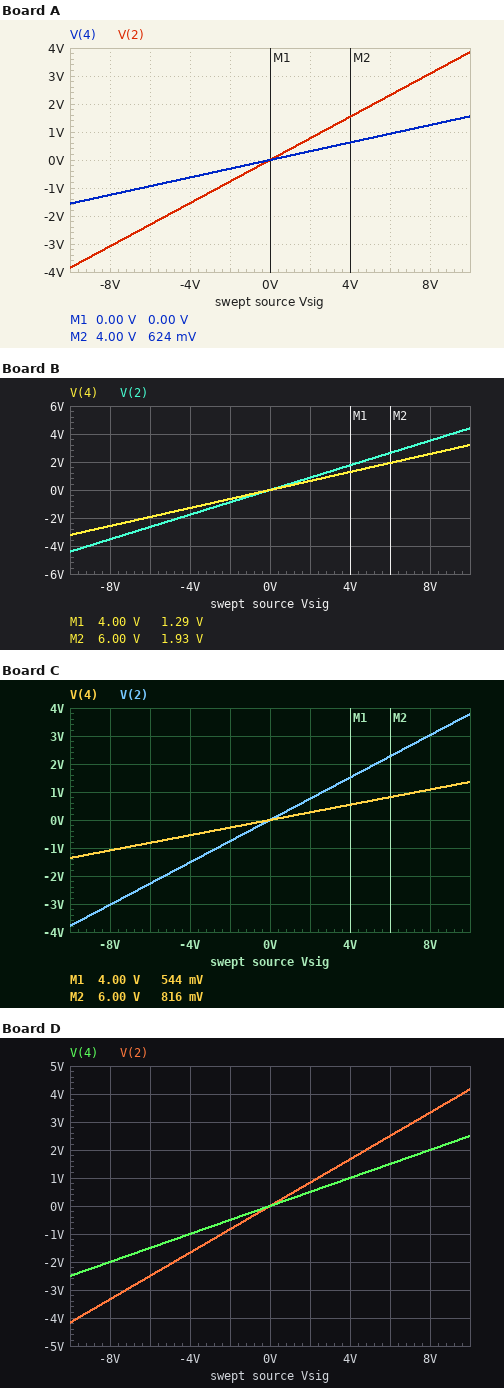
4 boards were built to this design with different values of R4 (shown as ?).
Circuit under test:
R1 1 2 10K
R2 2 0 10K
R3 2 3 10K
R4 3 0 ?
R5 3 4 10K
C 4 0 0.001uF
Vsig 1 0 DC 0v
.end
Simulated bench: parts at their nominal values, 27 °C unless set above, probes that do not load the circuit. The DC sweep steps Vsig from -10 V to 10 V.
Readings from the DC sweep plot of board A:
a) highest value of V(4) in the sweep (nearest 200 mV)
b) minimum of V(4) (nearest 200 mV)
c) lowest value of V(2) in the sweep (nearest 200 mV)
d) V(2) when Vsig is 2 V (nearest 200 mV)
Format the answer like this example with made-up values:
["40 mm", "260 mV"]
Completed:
["1.6 V", "-1.6 V", "-3.8 V", "800 mV"]
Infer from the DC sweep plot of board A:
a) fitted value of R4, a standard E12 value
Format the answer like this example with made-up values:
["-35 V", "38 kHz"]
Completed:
["6.8 kΩ"]
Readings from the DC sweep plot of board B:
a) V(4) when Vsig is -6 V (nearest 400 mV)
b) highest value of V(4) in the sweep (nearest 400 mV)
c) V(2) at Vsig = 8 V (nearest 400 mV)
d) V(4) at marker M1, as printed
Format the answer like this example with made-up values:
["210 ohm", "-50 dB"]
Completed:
["-2.0 V", "3.2 V", "3.6 V", "1.29 V"]
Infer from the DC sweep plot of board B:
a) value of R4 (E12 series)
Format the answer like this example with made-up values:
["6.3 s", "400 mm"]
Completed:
["27 kΩ"]
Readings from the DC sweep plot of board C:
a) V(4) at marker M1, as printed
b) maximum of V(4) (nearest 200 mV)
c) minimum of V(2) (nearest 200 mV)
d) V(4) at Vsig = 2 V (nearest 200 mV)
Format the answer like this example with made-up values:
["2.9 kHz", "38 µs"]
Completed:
["544 mV", "1.4 V", "-3.8 V", "200 mV"]
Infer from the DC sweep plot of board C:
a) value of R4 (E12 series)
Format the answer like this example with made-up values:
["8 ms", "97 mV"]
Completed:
["5.6 kΩ"]
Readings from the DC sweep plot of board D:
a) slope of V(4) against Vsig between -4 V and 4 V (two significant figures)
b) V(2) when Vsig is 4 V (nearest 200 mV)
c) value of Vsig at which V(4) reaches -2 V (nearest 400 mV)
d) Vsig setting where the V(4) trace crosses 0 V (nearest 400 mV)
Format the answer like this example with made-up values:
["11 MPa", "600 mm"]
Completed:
["0.25 V/V", "1.6 V", "-8.0 V", "0 V"]
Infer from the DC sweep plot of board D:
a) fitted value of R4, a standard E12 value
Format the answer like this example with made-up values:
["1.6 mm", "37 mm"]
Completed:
["15 kΩ"]
